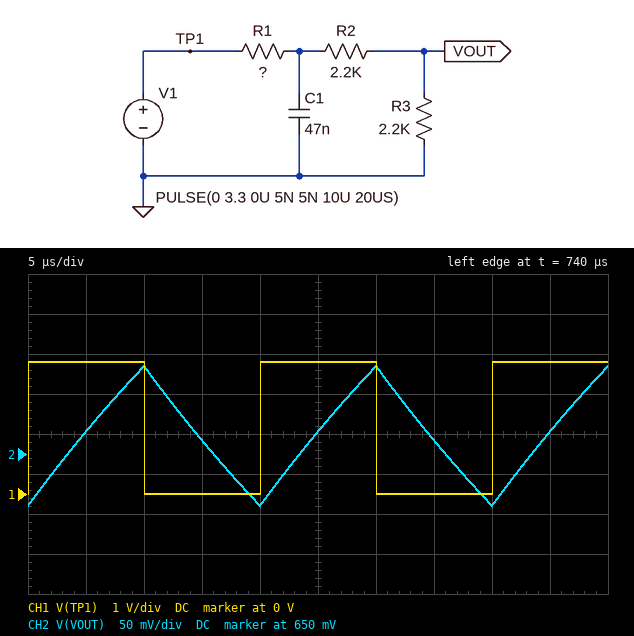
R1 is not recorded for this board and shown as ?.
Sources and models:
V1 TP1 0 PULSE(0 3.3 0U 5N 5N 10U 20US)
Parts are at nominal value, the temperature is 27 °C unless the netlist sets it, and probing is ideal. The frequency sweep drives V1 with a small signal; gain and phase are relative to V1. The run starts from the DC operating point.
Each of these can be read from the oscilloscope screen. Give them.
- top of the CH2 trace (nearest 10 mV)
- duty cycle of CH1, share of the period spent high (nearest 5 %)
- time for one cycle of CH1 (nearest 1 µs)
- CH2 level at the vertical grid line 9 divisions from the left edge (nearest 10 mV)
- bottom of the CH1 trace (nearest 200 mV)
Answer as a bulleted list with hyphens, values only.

- 760 mV
- 50 %
- 20 µs
- 680 mV
- 0 V
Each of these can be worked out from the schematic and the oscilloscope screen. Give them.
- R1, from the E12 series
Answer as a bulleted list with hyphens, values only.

- 1 kΩ
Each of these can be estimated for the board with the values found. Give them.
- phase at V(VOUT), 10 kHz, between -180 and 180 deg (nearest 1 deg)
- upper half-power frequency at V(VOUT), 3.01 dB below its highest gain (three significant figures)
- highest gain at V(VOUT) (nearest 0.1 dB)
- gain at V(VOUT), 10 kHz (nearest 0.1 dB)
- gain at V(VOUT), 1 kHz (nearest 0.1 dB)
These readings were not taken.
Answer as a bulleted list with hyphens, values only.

- -67 deg
- 4.16 kHz
- -7.8 dB
- -16.1 dB
- -8.0 dB
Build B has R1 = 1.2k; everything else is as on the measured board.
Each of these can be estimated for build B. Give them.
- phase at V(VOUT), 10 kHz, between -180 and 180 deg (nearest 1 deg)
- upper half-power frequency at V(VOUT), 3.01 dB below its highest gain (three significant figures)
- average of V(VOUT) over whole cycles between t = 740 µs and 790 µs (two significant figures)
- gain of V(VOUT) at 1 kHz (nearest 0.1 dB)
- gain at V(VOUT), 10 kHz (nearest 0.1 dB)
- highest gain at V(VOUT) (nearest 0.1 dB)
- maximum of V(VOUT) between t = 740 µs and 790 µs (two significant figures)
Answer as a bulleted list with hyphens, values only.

- -70 deg
- 3.59 kHz
- 650 mV
- -8.4 dB
- -17.5 dB
- -8.1 dB
- 720 mV
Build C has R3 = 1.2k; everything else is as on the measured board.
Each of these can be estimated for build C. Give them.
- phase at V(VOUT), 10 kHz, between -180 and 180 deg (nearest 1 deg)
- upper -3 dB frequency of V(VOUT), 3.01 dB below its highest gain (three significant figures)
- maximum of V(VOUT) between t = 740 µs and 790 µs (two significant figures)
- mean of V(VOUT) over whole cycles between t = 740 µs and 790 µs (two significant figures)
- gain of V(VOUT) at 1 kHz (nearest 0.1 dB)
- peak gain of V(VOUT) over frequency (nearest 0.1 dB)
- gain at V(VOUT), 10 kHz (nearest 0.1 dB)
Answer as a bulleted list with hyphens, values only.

- -66 deg
- 4.38 kHz
- 510 mV
- 450 mV
- -11.5 dB
- -11.3 dB
- -19.2 dB
